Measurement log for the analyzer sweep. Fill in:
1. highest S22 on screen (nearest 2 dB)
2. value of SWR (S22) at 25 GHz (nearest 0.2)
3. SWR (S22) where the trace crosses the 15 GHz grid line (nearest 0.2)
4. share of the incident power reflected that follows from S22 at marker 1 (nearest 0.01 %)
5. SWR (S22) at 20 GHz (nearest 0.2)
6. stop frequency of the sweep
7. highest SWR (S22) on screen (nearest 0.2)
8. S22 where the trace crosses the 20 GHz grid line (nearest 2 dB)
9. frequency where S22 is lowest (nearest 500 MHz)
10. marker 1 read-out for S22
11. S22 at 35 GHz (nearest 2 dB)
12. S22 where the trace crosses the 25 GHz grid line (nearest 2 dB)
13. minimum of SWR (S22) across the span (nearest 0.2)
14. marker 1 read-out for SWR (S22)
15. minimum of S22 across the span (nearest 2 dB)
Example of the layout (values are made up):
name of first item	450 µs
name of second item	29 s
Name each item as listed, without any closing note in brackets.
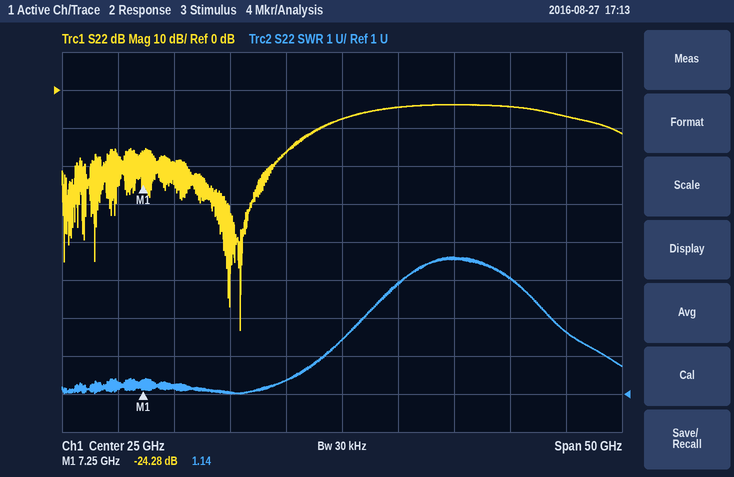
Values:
highest S22 on screen	-4 dB
value of SWR (S22) at 25 GHz	2.4
SWR (S22) where the trace crosses the 15 GHz grid line	1.0
share of the incident power reflected that follows from S22 at marker 1	0.37 %
SWR (S22) at 20 GHz	1.4
stop frequency of the sweep	50 GHz
highest SWR (S22) on screen	4.6
S22 where the trace crosses the 20 GHz grid line	-16 dB
frequency where S22 is lowest	16.0 GHz
marker 1 read-out for S22	-24.28 dB
S22 at 35 GHz	-4 dB
S22 where the trace crosses the 25 GHz grid line	-8 dB
minimum of SWR (S22) across the span	1.0
marker 1 read-out for SWR	1.14
minimum of S22 across the span	-64 dB
